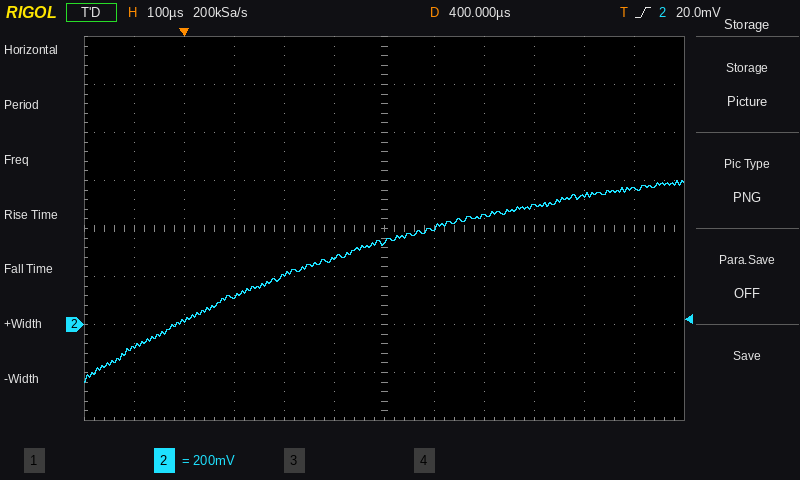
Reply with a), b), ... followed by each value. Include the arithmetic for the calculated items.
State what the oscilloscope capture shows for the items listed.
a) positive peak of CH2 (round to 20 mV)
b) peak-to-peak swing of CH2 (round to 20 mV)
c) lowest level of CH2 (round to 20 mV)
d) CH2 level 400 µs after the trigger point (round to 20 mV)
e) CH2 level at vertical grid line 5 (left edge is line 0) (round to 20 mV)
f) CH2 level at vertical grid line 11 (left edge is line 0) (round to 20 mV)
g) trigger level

a) 600 mV
b) 600 mV − (-240 mV) = 840 mV
c) -240 mV
d) 340 mV
e) 280 mV
f) 560 mV
g) 20.0 mV
